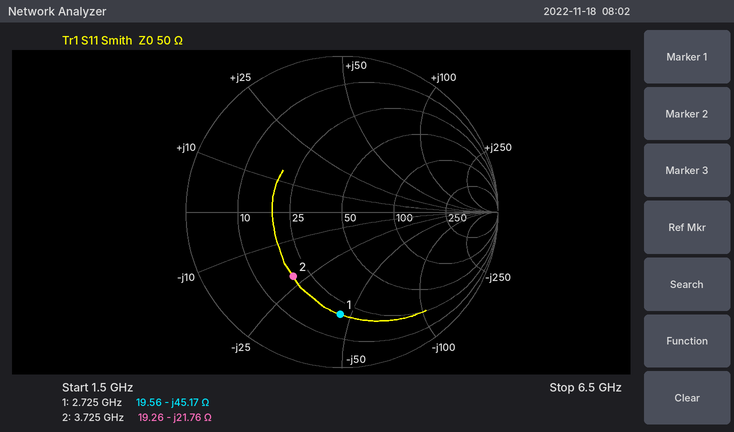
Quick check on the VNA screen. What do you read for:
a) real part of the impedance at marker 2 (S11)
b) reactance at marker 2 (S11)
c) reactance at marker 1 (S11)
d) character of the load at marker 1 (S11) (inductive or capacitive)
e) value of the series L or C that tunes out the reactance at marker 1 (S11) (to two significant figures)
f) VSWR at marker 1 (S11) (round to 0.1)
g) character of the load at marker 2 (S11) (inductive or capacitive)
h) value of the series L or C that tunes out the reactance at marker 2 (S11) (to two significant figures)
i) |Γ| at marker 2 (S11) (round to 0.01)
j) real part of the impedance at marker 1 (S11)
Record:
19.26 Ω
-21.76 Ω
-45.17 Ω
capacitive
2.6 nH
4.8
capacitive
930 pH
0.52
19.56 Ω
